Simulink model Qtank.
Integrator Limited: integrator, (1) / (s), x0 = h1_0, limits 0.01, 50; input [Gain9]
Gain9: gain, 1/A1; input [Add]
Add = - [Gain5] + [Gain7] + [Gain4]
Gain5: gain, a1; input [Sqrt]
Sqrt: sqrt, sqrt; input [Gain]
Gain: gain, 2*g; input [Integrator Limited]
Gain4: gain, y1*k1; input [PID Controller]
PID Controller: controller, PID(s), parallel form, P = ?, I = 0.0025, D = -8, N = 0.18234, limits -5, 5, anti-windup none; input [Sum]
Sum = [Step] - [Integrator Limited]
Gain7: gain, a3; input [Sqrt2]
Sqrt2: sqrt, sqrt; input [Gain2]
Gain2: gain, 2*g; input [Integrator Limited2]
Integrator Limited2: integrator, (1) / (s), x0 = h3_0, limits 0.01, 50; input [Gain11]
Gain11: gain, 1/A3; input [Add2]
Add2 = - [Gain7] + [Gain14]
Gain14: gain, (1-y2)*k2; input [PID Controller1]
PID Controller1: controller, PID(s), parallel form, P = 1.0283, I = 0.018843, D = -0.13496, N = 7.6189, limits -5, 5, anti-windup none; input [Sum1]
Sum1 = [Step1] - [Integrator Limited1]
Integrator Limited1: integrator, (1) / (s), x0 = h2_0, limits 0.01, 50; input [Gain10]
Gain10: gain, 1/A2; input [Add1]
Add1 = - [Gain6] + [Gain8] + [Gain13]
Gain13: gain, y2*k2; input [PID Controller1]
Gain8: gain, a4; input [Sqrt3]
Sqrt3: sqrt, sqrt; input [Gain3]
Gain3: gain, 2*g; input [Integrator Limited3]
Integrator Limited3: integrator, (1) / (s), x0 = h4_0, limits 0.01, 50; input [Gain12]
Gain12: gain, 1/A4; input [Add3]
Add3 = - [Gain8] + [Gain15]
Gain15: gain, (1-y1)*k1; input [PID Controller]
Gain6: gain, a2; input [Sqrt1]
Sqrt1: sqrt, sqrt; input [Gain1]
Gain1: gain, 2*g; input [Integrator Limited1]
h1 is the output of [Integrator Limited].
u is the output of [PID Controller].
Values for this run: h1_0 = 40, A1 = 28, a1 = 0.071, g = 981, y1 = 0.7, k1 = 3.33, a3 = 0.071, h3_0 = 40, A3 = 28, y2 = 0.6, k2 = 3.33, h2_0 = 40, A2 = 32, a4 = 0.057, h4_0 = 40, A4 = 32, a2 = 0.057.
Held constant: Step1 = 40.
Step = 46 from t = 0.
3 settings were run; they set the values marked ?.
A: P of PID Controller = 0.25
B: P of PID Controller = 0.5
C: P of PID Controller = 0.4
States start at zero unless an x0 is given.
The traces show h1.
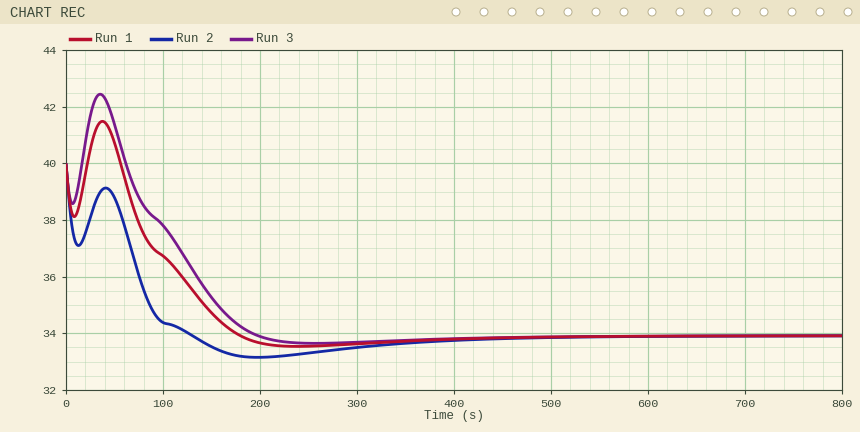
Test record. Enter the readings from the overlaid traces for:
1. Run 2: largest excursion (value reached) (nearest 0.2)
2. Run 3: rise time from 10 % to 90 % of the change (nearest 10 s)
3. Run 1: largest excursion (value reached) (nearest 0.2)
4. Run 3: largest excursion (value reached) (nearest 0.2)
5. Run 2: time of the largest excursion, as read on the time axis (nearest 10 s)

33.2
170 s
33.6
33.6
200 s
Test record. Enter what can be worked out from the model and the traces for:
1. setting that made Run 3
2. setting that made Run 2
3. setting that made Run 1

B
A
C
